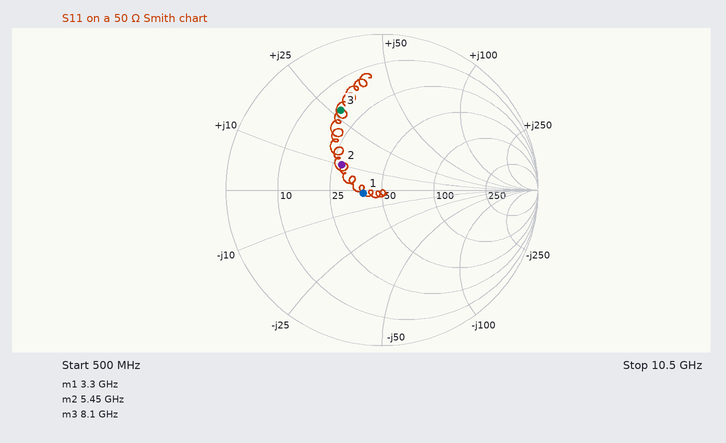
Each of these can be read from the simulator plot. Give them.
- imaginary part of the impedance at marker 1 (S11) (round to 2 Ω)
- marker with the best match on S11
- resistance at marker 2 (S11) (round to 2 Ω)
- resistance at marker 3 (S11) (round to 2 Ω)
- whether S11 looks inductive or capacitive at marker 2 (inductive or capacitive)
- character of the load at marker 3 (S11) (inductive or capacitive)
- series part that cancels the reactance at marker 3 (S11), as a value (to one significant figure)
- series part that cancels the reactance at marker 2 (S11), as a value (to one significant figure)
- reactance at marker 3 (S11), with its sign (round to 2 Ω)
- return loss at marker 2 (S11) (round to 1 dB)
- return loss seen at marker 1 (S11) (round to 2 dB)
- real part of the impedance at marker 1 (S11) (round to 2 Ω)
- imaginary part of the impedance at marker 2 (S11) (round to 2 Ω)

-2 Ω
marker 1
28 Ω
18 Ω
inductive
inductive
700 fF
3 pF
+28 Ω
10 dB
18 dB
40 Ω
+10 Ω
